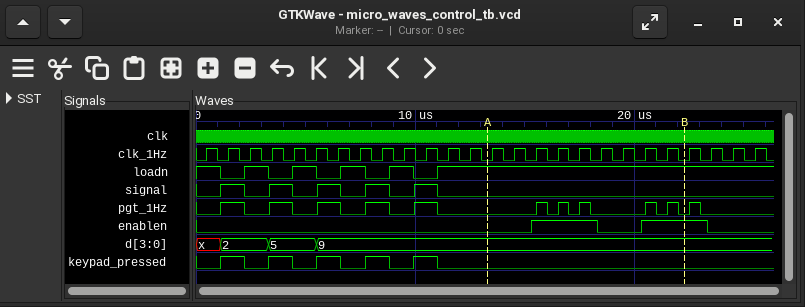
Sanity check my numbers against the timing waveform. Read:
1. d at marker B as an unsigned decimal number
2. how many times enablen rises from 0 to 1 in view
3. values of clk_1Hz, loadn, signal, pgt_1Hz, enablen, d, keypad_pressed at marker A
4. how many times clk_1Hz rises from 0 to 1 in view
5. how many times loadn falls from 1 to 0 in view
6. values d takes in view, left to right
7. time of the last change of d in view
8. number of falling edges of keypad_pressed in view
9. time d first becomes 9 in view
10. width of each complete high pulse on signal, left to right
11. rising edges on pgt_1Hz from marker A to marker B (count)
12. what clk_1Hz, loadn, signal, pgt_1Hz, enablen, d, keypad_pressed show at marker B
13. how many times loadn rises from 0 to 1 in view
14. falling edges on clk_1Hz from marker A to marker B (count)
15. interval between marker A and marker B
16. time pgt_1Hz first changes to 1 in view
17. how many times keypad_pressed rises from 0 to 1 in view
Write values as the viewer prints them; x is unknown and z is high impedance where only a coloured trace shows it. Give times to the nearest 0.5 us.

9
2
clk_1Hz=0, loadn=1, signal=0, pgt_1Hz=0, enablen=0, d=9, keypad_pressed=0
26
5
x, 2, 5, 9
5.5 us
5
5.5 us
1 us, 1 us, 1 us, 1 us, 1 us
5
clk_1Hz=0, loadn=1, signal=0, pgt_1Hz=0, enablen=1, d=9, keypad_pressed=0
5
9
9 us
1 us
5
